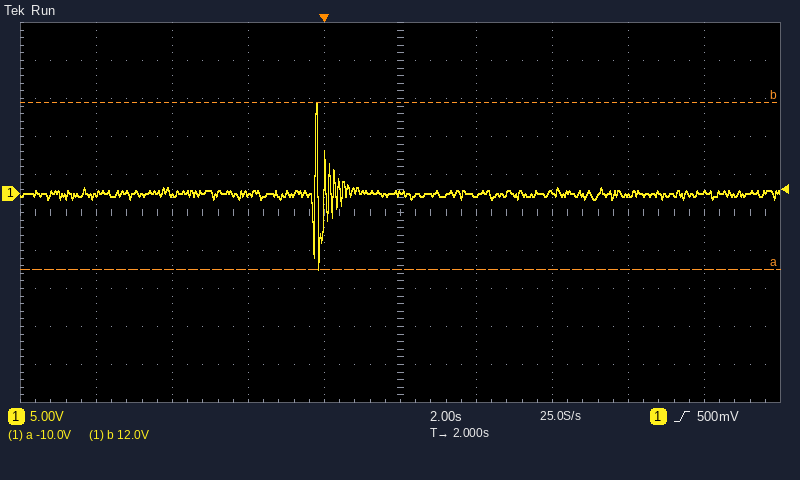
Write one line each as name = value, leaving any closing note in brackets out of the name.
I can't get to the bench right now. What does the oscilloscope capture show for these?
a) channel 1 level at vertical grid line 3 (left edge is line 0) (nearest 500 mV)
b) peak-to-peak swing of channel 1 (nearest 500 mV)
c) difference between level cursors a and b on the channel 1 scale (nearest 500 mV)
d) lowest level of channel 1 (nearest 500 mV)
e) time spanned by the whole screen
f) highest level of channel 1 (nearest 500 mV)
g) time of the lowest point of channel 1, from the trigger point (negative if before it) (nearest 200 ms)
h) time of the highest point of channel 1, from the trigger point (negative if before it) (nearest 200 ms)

channel 1 level at vertical grid line 3 (left edge is line 0) = 0.0 V
peak-to-peak swing of channel 1 = 22.0 V
difference between level cursors a and b on the channel 1 scale = 22.0 V
lowest level of channel 1 = -10.0 V
time spanned by the whole screen = 20 s
highest level of channel 1 = 12.0 V
time of the lowest point of channel 1, from the trigger point (negative if before it) = -200 ms
time of the highest point of channel 1, from the trigger point (negative if before it) = -200 ms
